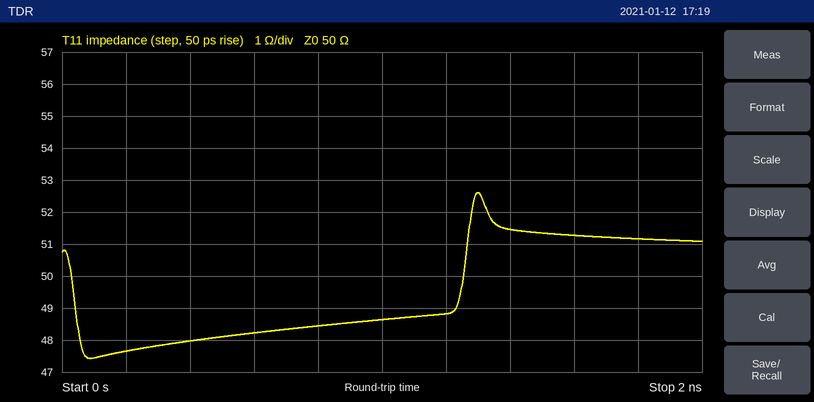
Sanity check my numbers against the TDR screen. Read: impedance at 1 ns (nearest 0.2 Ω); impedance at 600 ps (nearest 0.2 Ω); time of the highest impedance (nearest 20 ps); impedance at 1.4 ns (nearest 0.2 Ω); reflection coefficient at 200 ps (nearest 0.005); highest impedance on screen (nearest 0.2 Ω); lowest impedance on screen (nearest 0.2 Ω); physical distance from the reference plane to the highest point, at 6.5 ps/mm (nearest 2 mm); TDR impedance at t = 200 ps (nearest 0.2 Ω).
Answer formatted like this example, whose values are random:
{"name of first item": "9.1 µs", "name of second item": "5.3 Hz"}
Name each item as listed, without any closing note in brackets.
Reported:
{"impedance at 1 ns": "48.6 Ω", "impedance at 600 ps": "48.2 Ω", "time of the highest impedance": "1.30 ns", "impedance at 1.4 ns": "51.4 Ω", "reflection coefficient at 200 ps": "-0.025", "highest impedance on screen": "52.6 Ω", "lowest impedance on screen": "47.4 Ω", "physical distance from the reference plane to the highest point, at 6.5 ps/mm": "100 mm", "TDR impedance at t = 200 ps": "47.6 Ω"}
